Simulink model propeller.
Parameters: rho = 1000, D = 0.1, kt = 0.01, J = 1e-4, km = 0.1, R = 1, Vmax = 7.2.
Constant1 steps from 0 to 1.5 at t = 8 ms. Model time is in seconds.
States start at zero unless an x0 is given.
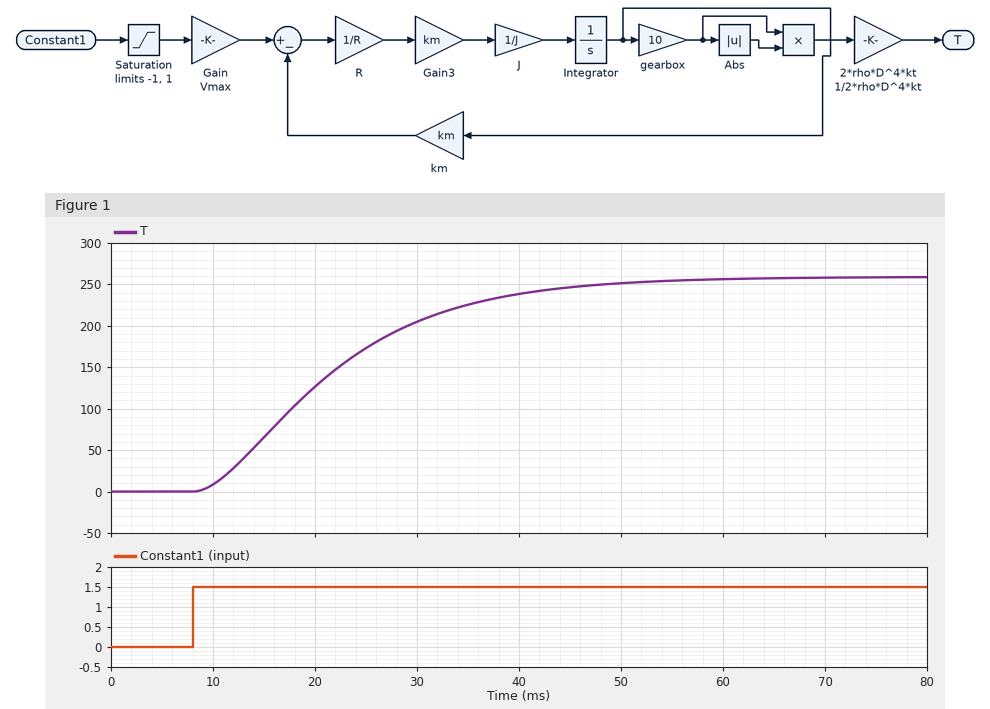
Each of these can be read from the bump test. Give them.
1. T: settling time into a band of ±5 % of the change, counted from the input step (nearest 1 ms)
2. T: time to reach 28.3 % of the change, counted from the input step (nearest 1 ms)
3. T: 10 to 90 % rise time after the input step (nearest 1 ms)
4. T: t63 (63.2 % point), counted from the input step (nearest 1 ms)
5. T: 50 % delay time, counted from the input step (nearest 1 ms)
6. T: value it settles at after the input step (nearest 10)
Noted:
37 ms
8 ms
26 ms
16 ms
12 ms
260
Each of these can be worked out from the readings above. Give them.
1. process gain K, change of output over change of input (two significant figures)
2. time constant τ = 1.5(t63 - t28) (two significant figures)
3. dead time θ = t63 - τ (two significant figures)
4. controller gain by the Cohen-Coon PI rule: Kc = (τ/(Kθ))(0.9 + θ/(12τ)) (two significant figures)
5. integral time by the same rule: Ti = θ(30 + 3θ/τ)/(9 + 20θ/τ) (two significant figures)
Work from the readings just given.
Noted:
170
12 ms
4.0 ms
0.016
7.9 ms
